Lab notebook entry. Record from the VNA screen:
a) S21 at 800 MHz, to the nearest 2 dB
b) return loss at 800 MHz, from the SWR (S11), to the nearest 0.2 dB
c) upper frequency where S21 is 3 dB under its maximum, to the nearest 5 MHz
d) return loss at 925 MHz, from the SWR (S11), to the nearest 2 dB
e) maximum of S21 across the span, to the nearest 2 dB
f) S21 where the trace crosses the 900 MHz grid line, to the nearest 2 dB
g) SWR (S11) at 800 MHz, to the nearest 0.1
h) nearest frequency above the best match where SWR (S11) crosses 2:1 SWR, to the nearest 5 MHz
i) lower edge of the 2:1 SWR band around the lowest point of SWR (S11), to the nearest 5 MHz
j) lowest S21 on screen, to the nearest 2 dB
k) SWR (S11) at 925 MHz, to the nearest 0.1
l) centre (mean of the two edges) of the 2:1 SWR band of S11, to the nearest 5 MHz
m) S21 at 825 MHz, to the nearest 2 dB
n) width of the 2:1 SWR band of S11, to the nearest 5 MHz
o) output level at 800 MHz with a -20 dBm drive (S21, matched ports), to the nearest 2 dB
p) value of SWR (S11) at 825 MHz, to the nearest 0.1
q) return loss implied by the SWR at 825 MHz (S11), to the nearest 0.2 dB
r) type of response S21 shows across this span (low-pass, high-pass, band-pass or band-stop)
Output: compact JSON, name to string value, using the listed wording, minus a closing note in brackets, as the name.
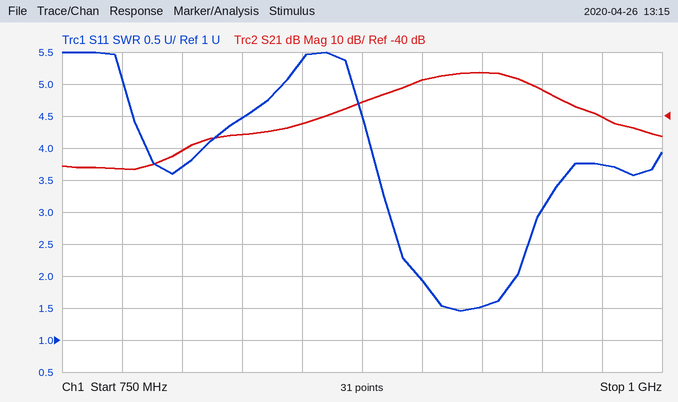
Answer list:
{"S21 at 800 MHz, to the nearest 2 dB": "-50 dB", "return loss at 800 MHz, from the SWR (S11), to the nearest 0.2 dB": "4.8 dB", "upper frequency where S21 is 3 dB under its maximum, to the nearest 5 MHz": "945 MHz", "return loss at 925 MHz, from the SWR (S11), to the nearest 2 dB": "14 dB", "maximum of S21 across the span, to the nearest 2 dB": "-26 dB", "S21 where the trace crosses the 900 MHz grid line, to the nearest 2 dB": "-28 dB", "SWR (S11) at 800 MHz, to the nearest 0.1": "3.7", "nearest frequency above the best match where SWR (S11) crosses 2:1 SWR, to the nearest 5 MHz": "940 MHz", "lower edge of the 2:1 SWR band around the lowest point of SWR (S11), to the nearest 5 MHz": "900 MHz", "lowest S21 on screen, to the nearest 2 dB": "-56 dB", "SWR (S11) at 925 MHz, to the nearest 0.1": "1.5", "centre (mean of the two edges) of the 2:1 SWR band of S11, to the nearest 5 MHz": "920 MHz", "S21 at 825 MHz, to the nearest 2 dB": "-46 dB", "width of the 2:1 SWR band of S11, to the nearest 5 MHz": "40 MHz", "output level at 800 MHz with a -20 dBm drive (S21, matched ports), to the nearest 2 dB": "-70 dBm", "value of SWR (S11) at 825 MHz, to the nearest 0.1": "4.5", "return loss implied by the SWR at 825 MHz (S11), to the nearest 0.2 dB": "4.0 dB", "type of response S21 shows across this span": "band-pass"}
